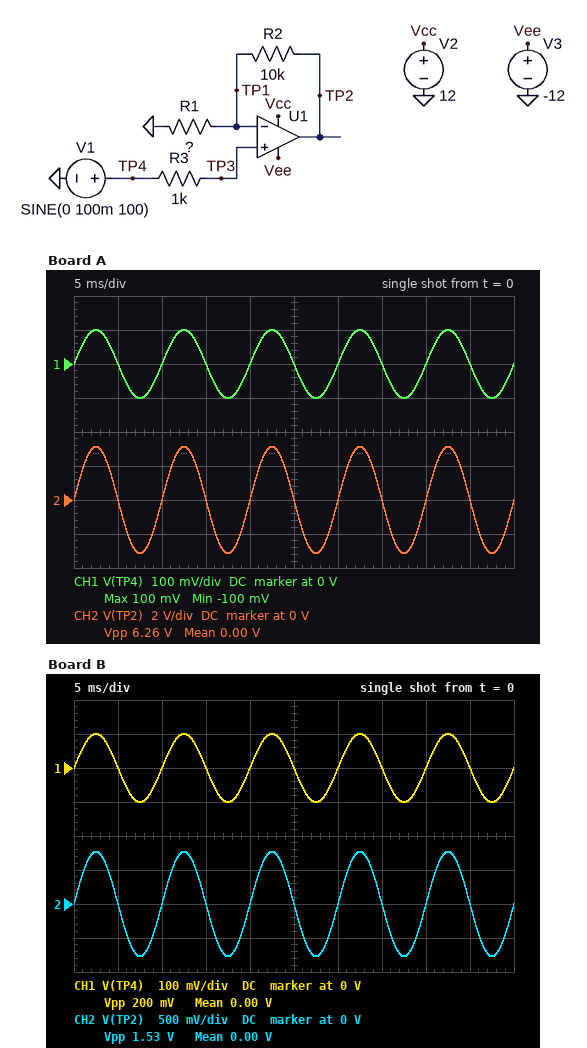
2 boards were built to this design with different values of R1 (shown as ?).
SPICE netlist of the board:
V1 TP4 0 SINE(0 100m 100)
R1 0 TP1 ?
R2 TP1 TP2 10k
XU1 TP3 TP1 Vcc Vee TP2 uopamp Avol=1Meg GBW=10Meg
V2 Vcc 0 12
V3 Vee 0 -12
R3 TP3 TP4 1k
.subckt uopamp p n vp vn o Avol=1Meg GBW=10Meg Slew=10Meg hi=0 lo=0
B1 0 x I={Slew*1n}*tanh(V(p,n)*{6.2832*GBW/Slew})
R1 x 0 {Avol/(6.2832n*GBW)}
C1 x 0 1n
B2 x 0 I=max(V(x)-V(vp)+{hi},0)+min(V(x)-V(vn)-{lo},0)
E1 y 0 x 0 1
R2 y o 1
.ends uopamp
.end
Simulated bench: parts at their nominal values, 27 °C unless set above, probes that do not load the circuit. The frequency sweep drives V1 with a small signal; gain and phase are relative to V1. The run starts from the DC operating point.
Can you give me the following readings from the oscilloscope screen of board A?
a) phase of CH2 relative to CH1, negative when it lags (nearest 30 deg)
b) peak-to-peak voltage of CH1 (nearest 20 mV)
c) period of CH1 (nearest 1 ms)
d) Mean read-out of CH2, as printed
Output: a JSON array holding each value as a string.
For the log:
["0 deg", "200 mV", "10 ms", "0.00 V"]
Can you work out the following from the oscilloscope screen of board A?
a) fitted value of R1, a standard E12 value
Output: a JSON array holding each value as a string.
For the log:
["330 Ω"]
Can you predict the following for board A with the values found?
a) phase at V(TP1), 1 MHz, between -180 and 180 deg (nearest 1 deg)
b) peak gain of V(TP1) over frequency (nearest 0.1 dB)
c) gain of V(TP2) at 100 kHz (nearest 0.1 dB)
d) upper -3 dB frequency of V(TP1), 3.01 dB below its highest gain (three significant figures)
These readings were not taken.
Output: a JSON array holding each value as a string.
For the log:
["-72 deg", "0 dB", "29.5 dB", "319 kHz"]
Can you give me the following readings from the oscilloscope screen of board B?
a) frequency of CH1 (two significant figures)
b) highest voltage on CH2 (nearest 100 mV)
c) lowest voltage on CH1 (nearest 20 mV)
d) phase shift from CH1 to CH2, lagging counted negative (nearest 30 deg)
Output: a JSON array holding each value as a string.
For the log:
["100 Hz", "800 mV", "-100 mV", "0 deg"]
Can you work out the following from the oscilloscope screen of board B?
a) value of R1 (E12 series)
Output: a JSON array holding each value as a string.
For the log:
["1.5 kΩ"]
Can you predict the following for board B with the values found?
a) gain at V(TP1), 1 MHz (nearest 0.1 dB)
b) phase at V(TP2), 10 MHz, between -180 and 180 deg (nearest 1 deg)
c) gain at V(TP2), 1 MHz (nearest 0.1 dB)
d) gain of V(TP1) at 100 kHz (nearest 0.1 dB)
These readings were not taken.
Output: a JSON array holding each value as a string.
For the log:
["-2.0 dB", "-83 deg", "15.7 dB", "0 dB"]
